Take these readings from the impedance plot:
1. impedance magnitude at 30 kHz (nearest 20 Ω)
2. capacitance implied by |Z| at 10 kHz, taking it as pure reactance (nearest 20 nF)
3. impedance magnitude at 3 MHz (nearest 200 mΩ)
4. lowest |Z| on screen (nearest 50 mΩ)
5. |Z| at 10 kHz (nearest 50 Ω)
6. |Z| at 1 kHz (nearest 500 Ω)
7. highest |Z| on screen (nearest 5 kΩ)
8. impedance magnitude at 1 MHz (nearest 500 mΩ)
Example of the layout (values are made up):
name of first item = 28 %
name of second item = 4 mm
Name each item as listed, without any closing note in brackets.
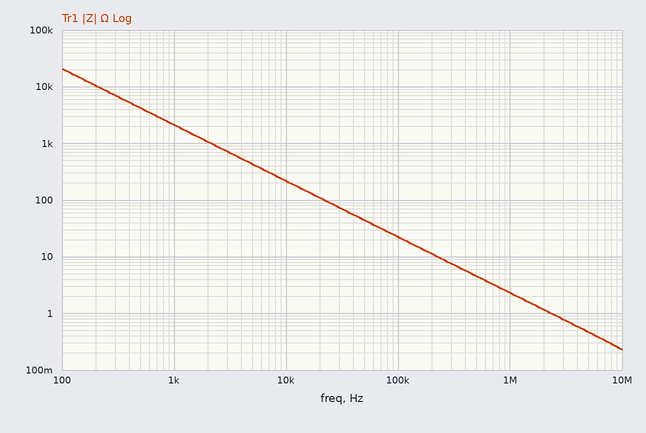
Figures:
impedance magnitude at 30 kHz = 80 Ω
capacitance implied by |Z| at 10 kHz, taking it as pure reactance = 80 nF
impedance magnitude at 3 MHz = 800 mΩ
lowest |Z| on screen = 250 mΩ
|Z| at 10 kHz = 200 Ω
|Z| at 1 kHz = 2.0 kΩ
highest |Z| on screen = 20 kΩ
impedance magnitude at 1 MHz = 2.5 Ω
